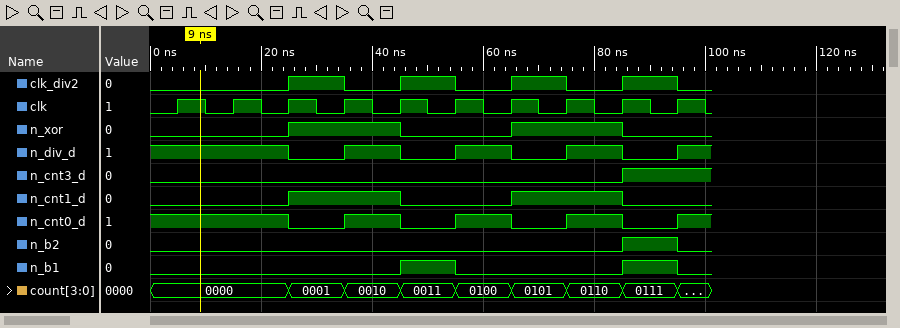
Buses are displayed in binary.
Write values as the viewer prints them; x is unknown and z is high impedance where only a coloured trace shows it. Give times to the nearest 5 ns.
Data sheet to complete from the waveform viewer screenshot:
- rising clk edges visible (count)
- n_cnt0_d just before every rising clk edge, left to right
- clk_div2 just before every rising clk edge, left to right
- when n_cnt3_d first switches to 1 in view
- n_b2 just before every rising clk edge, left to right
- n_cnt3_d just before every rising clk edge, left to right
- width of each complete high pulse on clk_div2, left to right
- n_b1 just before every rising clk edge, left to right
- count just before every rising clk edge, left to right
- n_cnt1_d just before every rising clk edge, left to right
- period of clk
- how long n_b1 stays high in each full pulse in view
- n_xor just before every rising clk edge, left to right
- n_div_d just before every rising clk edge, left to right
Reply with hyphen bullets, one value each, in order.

- 10
- 1 1 1 0 1 0 1 0 1 0
- 0 0 0 1 0 1 0 1 0 1
- 85 ns
- 0 0 0 0 0 0 0 0 0 1
- 0 0 0 0 0 0 0 0 0 1
- 10 ns, 10 ns, 10 ns, 10 ns
- 0 0 0 0 0 1 0 0 0 1
- 0000, 0000, 0000, 0001, 0010, 0011, 0100, 0101, 0110, 0111
- 0 0 0 1 1 0 0 1 1 0
- 10 ns
- 10 ns, 10 ns
- 0 0 0 1 1 0 0 1 1 0
- 1 1 1 0 1 0 1 0 1 0
